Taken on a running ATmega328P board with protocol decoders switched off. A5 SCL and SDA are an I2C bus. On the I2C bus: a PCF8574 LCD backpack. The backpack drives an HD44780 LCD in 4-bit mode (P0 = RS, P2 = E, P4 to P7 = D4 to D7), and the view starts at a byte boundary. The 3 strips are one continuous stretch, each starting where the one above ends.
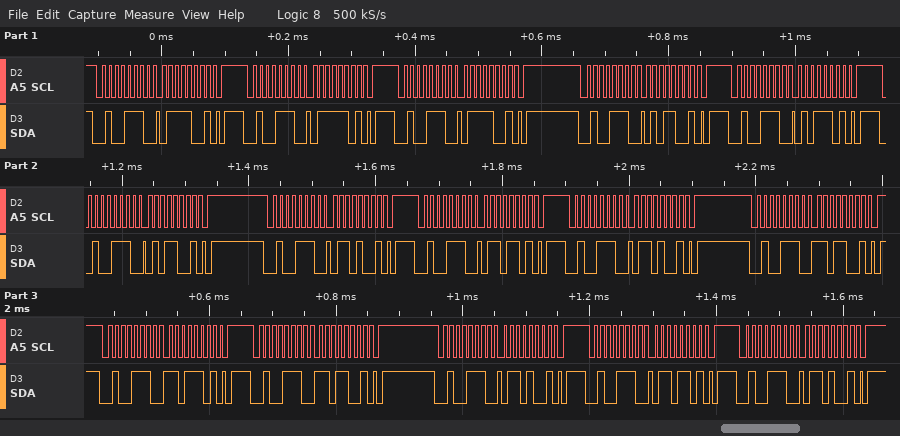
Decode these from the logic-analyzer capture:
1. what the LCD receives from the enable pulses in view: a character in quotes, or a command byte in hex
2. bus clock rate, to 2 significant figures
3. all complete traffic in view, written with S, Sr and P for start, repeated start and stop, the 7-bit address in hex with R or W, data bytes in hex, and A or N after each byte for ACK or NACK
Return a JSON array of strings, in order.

["'u' 'm'", "100 kHz", "S 27W A 79 A P S 27W A 7D A P S 27W A 79 A P S 27W A 59 A P S 27W A 5D A P S 27W A 59 A P S 27W A 69 A P S 27W A 6D A P S 27W A 69 A P S 27W A D9 A P S 27W A DD A P S 27W A D9 A P S 27W A 69 A P S 27W A 6D A P S 27W A 69 A P"]
